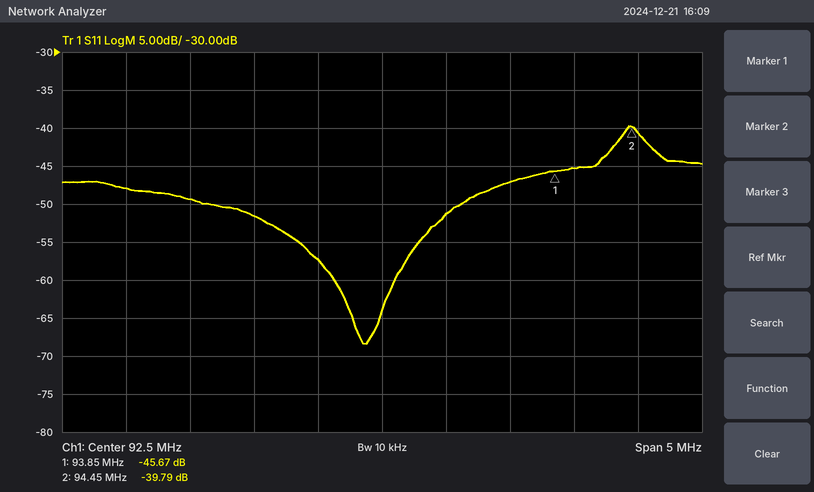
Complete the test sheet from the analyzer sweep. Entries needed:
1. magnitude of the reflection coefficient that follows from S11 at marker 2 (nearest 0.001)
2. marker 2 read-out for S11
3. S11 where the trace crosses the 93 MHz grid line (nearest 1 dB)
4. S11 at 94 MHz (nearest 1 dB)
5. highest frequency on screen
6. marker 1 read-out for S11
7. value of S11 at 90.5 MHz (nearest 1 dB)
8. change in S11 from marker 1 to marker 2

0.010
-39.79 dB
-51 dB
-45 dB
95 MHz
-45.67 dB
-48 dB
5.88 dB
